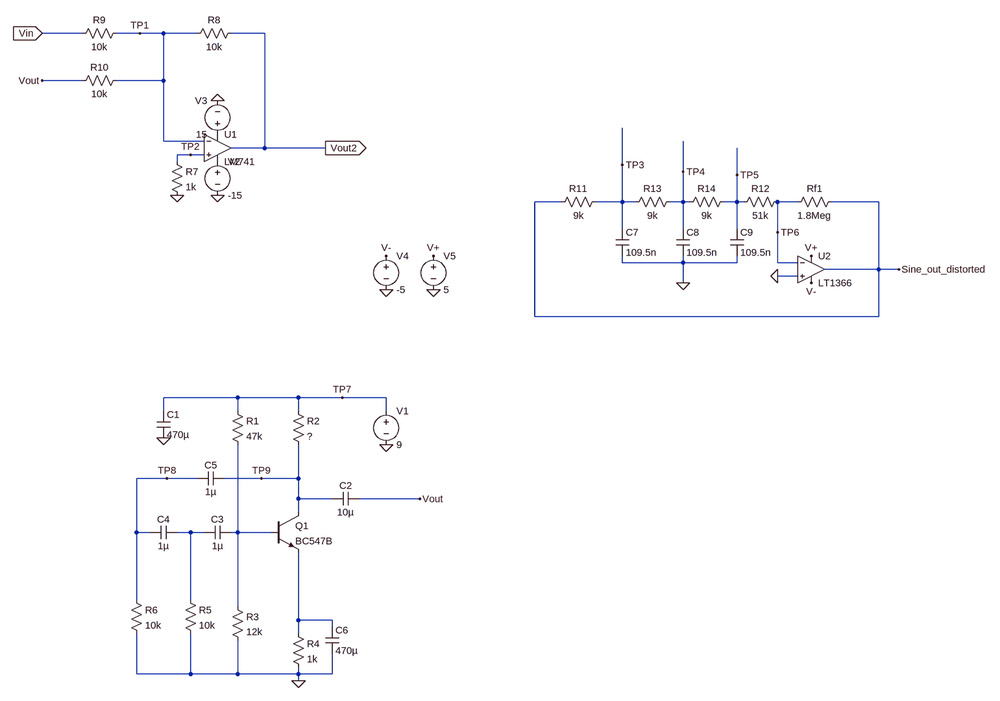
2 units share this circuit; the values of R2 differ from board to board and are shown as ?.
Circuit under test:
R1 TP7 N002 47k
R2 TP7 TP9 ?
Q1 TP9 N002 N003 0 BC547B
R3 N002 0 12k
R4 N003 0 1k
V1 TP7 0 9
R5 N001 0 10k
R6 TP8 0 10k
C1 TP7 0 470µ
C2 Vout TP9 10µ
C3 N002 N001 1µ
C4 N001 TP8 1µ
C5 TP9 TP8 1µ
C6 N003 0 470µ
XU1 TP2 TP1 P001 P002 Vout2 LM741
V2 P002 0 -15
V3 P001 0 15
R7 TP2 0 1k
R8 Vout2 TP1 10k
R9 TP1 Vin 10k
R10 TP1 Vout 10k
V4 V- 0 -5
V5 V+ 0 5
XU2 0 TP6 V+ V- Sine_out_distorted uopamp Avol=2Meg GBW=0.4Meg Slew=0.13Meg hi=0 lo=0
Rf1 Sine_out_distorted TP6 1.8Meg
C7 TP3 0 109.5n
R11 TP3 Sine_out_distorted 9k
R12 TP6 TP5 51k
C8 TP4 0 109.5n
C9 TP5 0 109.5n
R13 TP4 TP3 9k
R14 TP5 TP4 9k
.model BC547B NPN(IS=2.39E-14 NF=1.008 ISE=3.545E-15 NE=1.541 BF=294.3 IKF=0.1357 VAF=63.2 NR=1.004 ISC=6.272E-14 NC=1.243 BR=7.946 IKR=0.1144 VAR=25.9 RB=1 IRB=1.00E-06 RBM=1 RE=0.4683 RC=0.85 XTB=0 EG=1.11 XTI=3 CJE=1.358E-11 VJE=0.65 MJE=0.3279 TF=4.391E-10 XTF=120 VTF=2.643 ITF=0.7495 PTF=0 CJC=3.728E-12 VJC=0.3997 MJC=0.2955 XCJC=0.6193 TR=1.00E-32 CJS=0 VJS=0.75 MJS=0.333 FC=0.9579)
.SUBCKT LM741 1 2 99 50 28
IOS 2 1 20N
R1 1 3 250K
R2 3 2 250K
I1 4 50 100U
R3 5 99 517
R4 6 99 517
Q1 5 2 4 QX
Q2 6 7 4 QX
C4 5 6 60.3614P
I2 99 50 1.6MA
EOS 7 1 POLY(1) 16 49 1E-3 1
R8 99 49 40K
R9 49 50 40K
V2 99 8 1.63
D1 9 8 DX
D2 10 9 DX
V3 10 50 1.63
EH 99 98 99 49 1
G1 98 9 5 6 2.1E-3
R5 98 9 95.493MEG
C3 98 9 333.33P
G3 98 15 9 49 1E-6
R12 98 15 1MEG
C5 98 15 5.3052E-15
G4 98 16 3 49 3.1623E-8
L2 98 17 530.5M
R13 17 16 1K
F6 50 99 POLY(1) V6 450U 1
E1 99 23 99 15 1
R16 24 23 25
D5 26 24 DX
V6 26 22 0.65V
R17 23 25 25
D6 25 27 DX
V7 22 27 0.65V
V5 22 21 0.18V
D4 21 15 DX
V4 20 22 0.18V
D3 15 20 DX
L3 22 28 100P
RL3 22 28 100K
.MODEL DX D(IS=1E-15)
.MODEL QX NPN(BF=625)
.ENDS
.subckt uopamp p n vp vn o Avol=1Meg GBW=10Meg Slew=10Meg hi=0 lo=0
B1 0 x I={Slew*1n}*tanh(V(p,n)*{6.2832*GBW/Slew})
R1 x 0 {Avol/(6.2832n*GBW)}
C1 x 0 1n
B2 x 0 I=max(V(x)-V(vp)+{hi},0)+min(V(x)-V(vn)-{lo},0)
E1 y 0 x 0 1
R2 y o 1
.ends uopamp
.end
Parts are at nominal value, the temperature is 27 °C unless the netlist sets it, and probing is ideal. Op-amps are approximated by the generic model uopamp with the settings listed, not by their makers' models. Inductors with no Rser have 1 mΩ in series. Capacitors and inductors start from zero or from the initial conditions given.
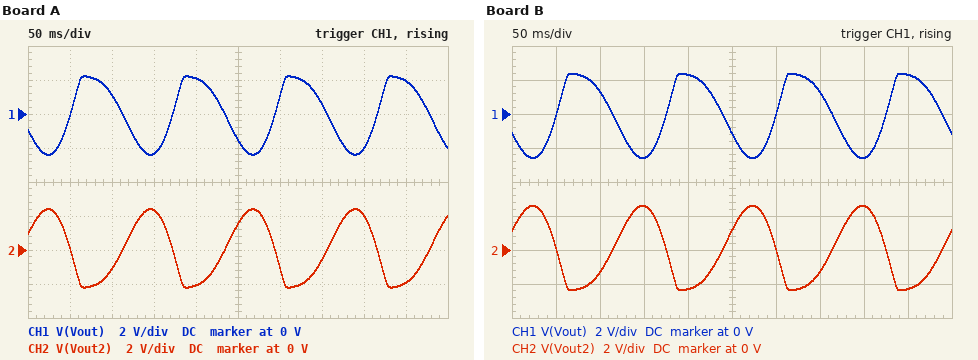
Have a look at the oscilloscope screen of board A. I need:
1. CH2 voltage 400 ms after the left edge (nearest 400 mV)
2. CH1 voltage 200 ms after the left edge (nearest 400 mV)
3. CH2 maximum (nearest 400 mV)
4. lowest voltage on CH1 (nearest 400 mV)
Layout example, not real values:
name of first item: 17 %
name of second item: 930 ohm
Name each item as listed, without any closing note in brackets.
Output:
CH2 voltage 400 ms after the left edge: 2.0 V
CH1 voltage 200 ms after the left edge: 2.0 V
CH2 maximum: 2.4 V
lowest voltage on CH1: -2.4 V
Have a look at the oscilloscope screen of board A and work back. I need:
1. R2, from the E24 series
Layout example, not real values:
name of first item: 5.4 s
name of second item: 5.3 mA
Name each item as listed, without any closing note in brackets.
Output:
R2, from the E24 series: 2.2 kΩ
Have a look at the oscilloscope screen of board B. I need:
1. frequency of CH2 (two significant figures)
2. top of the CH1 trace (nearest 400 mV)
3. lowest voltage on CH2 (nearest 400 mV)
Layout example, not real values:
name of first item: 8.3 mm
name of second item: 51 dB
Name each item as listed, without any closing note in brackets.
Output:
frequency of CH2: 8.0 Hz
top of the CH1 trace: 2.4 V
lowest voltage on CH2: -2.4 V
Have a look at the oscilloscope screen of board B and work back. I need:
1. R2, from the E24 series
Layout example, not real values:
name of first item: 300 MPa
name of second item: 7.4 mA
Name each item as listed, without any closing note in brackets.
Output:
R2, from the E24 series: 2.4 kΩ
